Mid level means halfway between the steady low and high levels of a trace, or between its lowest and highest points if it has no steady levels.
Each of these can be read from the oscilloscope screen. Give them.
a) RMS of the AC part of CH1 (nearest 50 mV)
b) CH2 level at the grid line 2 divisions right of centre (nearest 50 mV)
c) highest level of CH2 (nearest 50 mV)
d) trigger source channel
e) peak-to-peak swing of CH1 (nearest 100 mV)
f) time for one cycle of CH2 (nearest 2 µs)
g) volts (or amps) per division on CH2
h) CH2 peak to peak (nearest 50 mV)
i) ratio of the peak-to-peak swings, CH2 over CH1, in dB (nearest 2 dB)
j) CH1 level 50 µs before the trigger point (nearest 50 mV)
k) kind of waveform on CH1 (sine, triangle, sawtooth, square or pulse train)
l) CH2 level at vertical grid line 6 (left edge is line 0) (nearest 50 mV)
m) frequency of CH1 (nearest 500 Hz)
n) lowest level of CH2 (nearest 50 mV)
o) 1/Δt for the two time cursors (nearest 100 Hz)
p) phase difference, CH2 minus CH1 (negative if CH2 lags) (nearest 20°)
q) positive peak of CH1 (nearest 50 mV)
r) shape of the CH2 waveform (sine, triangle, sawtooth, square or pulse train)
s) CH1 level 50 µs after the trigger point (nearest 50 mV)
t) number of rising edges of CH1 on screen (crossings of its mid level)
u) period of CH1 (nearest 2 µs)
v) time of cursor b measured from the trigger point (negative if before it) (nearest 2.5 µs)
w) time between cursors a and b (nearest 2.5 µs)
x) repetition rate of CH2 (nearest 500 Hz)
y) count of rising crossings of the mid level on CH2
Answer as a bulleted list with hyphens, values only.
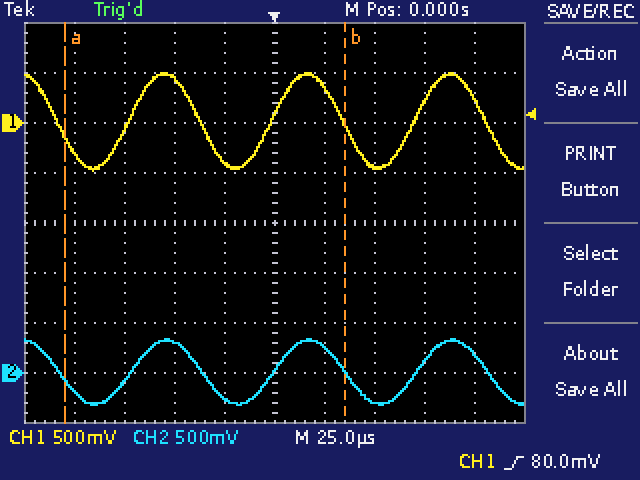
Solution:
- 350 mV
- -300 mV
- 350 mV
- CH1
- 1.00 V
- 72 µs
- 500 mV
- 650 mV
- -4 dB
- 450 mV
- sine
- 250 mV
- 14.0 kHz
- -300 mV
- 7.1 kHz
- 0°
- 500 mV
- sine
- -450 mV
- 3
- 72 µs
- +35.0 µs
- 140.0 µs
- 14.0 kHz
- 3
